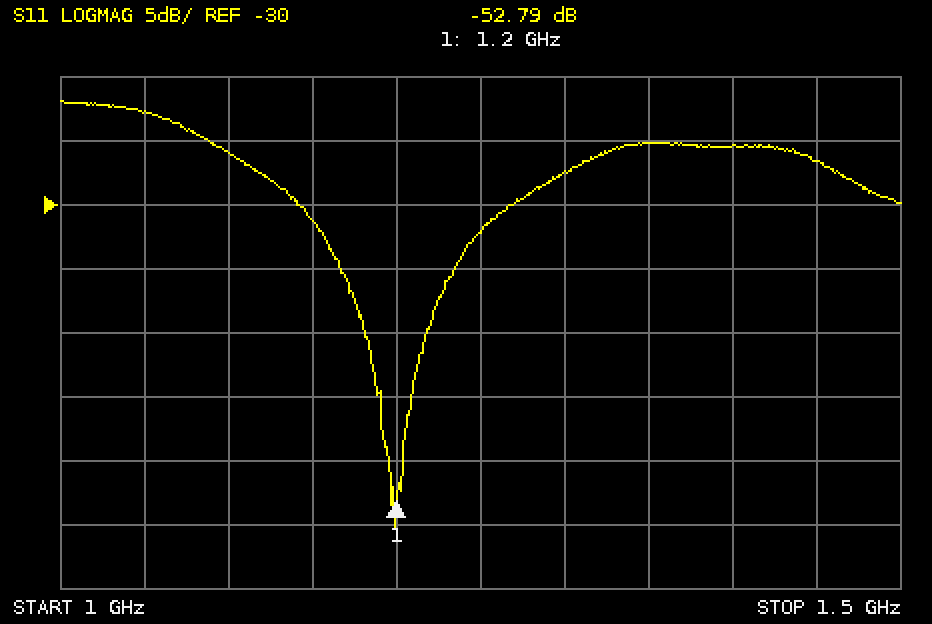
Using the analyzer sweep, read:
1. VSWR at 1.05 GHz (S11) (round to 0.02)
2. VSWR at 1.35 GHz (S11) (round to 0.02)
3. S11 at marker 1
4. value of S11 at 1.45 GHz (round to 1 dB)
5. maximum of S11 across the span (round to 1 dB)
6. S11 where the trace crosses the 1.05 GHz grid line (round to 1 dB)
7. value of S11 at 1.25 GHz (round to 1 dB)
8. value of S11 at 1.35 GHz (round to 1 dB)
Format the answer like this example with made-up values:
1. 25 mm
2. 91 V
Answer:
1. 1.16
2. 1.12
3. -52.79 dB
4. -27 dB
5. -22 dB
6. -23 dB
7. -32 dB
8. -25 dB
